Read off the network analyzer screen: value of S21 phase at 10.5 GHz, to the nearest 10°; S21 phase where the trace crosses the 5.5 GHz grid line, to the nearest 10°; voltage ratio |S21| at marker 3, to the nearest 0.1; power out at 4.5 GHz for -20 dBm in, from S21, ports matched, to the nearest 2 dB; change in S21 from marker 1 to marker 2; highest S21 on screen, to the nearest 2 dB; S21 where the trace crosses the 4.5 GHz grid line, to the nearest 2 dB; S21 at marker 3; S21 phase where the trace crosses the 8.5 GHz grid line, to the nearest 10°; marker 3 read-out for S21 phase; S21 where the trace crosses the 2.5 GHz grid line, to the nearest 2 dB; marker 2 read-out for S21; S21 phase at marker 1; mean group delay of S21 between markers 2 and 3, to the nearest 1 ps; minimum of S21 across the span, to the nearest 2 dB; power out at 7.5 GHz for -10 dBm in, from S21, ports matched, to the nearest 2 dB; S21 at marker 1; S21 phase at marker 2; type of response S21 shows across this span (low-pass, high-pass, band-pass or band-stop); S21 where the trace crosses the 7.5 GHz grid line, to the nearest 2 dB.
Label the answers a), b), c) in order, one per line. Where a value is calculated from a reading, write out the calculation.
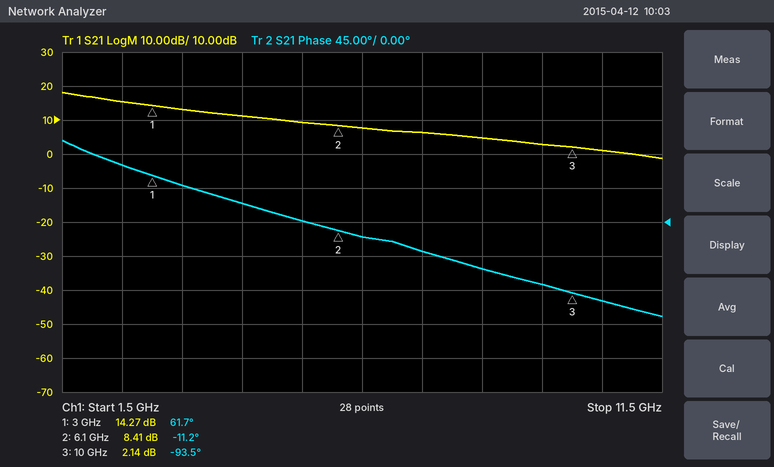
a) -100°
b) 0°
c) 10^(2.14/20) ≈ 1.3
d) -20 dBm + (12 dB) = -8 dBm
e) 8.41 − (14.27) = -5.86 dB
f) 18 dB
g) 12 dB
h) 2.14 dB
i) -60°
j) -93.5°
k) 16 dB
l) 8.41 dB
m) 61.7°
n) −(-93.5° − (-11.2°))/(360° × 3.9 GHz) ≈ 59 ps
o) -2 dB
p) -10 dBm + (6 dB) = -4 dBm
q) 14.27 dB
r) -11.2°
s) low-pass
t) 6 dB
